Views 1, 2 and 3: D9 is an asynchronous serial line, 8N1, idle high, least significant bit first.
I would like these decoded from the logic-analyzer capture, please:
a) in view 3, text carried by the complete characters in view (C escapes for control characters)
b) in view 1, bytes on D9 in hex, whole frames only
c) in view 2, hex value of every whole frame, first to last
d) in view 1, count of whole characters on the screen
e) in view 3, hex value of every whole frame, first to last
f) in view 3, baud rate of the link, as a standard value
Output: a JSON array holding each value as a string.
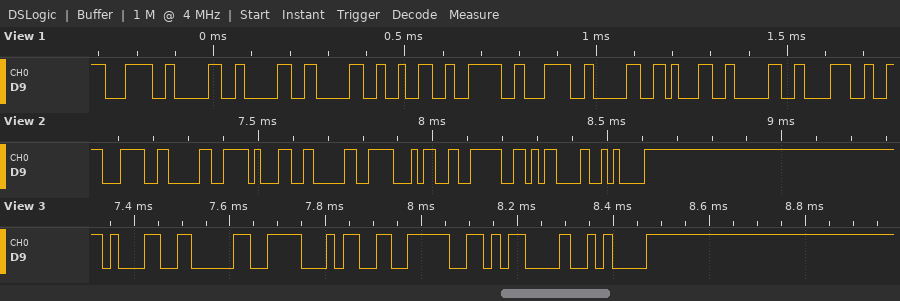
["\"104>\\r\\n\"", "0x3C 0x30 0x30 0x30 0x32 0x3E 0x3C 0x30 0x31 0x30 0x38", "0x3C 0x30 0x31 0x30 0x34 0x3E 0x0D 0x0A", "11", "31 30 34 3E 0D 0A", "57600 baud"]
